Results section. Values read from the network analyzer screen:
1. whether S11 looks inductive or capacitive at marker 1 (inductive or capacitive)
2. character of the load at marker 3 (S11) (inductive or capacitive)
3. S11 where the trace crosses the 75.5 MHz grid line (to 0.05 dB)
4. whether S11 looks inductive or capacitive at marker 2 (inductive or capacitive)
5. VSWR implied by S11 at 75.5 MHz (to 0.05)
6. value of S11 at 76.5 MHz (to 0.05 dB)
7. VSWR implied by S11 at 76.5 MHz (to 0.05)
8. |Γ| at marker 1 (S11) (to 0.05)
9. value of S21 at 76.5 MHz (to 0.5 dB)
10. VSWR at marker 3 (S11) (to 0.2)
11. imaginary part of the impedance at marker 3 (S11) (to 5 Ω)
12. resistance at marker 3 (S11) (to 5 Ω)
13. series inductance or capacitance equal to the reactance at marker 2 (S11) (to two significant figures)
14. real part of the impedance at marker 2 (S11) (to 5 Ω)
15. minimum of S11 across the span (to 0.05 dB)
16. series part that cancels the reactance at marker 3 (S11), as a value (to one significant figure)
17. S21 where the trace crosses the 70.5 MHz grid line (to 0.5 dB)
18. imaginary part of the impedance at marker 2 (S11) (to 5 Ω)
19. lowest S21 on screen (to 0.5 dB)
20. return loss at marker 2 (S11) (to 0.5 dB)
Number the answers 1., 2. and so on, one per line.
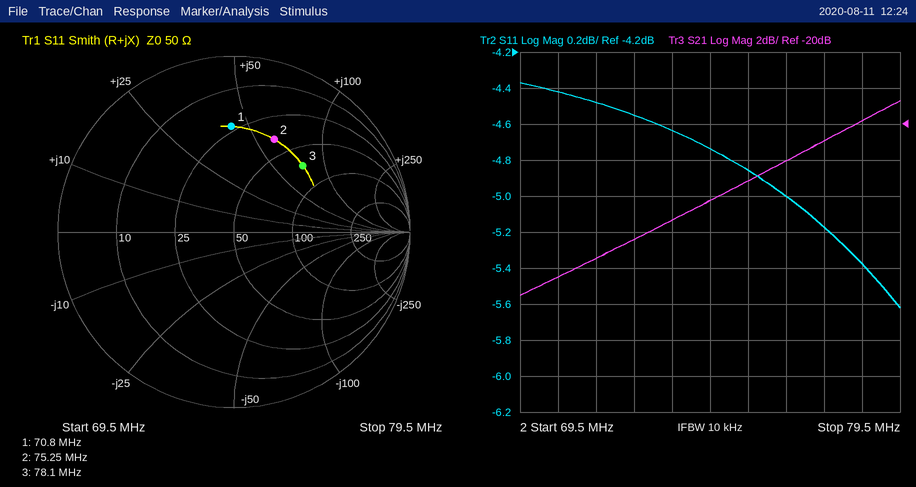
1. inductive
2. inductive
3. -4.85 dB
4. inductive
5. 3.65
6. -5.00 dB
7. 3.55
8. 0.60
9. -22.0 dB
10. 3.4
11. +75 Ω
12. 70 Ω
13. 130 nH
14. 40 Ω
15. -5.60 dB
16. 30 pF
17. -28.5 dB
18. +60 Ω
19. -29.5 dB
20. 5.0 dB
